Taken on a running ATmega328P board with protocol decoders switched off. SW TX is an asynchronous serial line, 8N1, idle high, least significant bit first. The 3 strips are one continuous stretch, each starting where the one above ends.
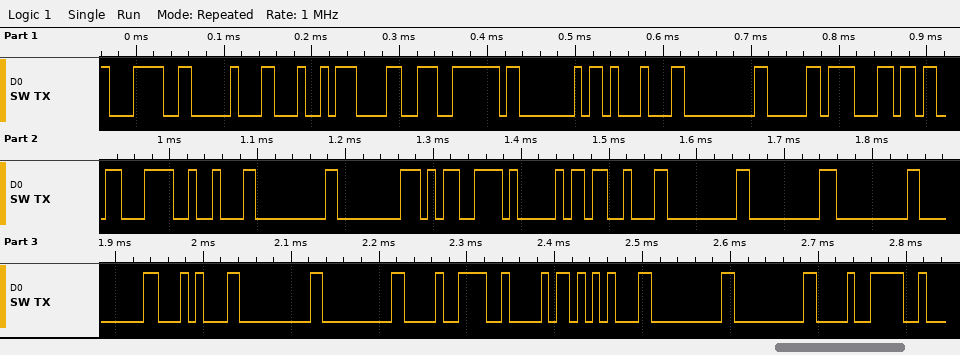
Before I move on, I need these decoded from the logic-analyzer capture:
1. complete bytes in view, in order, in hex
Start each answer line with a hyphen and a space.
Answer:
- 0x3C 0x10 0xA4 0x98 0x7E 0x40 0x11 0x00 0xB0 0x6C 0xC6 0x12 0x00 0x80 0xCD 0x41 0x13 0x00 0x00 0x00 0x00 0x14 0x00 0x00 0xC8 0x42 0x15 0x00 0x00 0xC8
